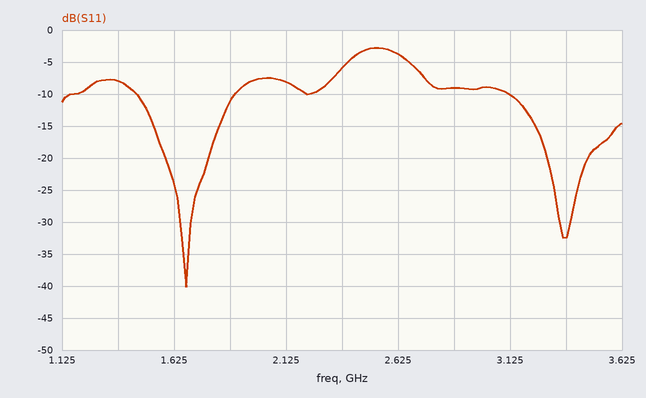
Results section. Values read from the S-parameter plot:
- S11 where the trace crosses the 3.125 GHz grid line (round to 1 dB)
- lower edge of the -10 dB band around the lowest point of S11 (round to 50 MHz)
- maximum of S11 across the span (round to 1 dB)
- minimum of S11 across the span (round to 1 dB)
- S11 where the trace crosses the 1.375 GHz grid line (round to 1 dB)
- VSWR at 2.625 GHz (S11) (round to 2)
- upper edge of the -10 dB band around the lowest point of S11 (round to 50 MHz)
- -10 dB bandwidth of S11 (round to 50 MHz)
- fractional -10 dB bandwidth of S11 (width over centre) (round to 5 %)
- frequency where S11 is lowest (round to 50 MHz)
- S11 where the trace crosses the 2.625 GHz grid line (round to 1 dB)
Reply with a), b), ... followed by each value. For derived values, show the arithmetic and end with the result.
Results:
a) -10 dB
b) 1.45 GHz
c) -3 dB
d) -40 dB
e) -8 dB
f) |Γ| = 10^(-4/20) = 0.6310; VSWR = (1 + 0.6310)/(1 − 0.6310) ≈ 4
g) 1.90 GHz
h) 1.90 GHz − 1.45 GHz = 450 MHz
i) 450 MHz / 1.675 GHz ≈ 26.9 %, so 25 % to the nearest 5 %
j) 1.70 GHz
k) -4 dB
